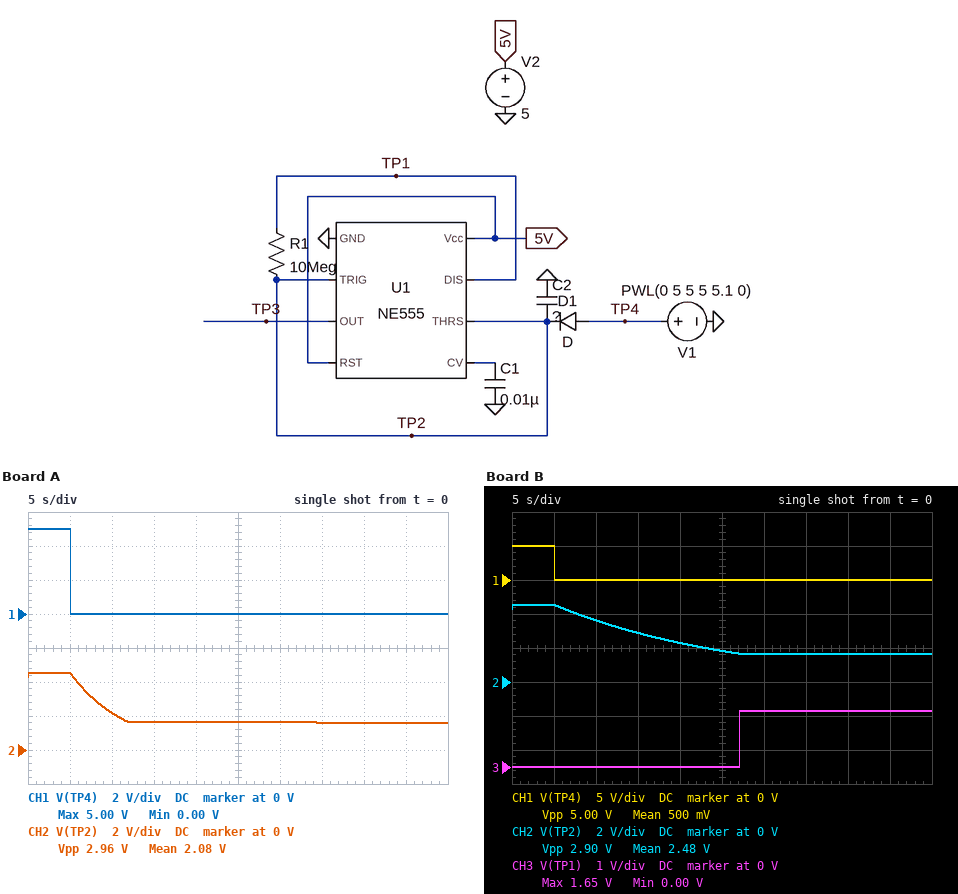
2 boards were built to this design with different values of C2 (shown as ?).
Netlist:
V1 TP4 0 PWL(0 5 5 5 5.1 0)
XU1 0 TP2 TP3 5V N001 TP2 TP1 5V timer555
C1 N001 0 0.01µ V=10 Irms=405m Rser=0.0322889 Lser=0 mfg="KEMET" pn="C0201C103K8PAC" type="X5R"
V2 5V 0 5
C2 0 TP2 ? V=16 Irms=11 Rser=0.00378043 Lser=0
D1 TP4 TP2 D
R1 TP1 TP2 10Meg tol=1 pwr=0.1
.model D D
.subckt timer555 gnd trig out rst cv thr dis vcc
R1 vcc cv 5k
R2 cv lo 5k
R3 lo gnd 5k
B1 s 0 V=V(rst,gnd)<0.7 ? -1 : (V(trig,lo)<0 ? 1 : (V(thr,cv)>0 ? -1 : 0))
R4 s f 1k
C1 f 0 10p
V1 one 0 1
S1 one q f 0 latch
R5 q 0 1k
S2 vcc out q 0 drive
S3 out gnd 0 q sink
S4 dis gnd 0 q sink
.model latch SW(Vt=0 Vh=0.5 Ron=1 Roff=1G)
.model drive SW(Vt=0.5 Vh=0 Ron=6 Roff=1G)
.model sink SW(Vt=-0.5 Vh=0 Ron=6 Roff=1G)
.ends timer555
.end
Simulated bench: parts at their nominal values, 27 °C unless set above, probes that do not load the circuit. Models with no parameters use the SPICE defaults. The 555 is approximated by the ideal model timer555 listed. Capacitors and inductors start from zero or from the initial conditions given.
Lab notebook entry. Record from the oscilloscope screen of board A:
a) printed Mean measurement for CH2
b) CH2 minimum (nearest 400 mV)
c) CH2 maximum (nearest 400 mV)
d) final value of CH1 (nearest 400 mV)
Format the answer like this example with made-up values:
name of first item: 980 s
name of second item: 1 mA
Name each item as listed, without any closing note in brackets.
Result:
printed Mean measurement for CH2: 2.08 V
CH2 minimum: 1.6 V
CH2 maximum: 4.4 V
final value of CH1: 0 V
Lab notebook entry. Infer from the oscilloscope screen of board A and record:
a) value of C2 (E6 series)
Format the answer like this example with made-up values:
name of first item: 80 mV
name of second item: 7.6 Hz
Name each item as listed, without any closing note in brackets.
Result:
value of C2: 680 nF
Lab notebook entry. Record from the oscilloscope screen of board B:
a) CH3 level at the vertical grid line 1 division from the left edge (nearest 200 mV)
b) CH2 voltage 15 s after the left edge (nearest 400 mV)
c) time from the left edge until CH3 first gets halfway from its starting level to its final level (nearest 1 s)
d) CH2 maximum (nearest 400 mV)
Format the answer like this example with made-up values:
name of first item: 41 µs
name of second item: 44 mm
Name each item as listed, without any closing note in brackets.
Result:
CH3 level at the vertical grid line 1 division from the left edge: 0 V
CH2 voltage 15 s after the left edge: 2.8 V
time from the left edge until CH3 first gets halfway from its starting level to its final level: 27 s
CH2 maximum: 4.4 V
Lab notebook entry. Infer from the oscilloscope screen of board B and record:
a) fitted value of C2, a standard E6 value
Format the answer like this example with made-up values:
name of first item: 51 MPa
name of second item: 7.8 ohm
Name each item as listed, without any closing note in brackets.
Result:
fitted value of C2, a standard E6 value: 2.2 µF
